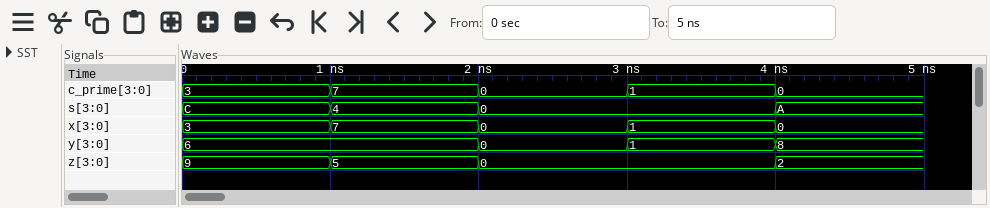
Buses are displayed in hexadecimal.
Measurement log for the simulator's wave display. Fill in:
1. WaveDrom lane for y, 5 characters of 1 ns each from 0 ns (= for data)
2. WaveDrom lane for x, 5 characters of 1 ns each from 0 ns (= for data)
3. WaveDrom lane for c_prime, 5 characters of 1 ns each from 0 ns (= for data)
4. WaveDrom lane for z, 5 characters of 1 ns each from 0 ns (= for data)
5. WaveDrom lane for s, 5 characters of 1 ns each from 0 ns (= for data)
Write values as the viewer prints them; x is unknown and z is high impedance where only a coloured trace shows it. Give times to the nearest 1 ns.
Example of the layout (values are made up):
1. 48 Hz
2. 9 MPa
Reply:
1. {name: 'y', wave: '=.===', data: '6 0 1 8'}
2. {name: 'x', wave: '=====', data: '3 7 0 1 0'}
3. {name: 'c_prime', wave: '=====', data: '3 7 0 1 0'}
4. {name: 'z', wave: '===.=', data: '9 5 0 2'}
5. {name: 's', wave: '===.=', data: 'C 4 0 A'}
